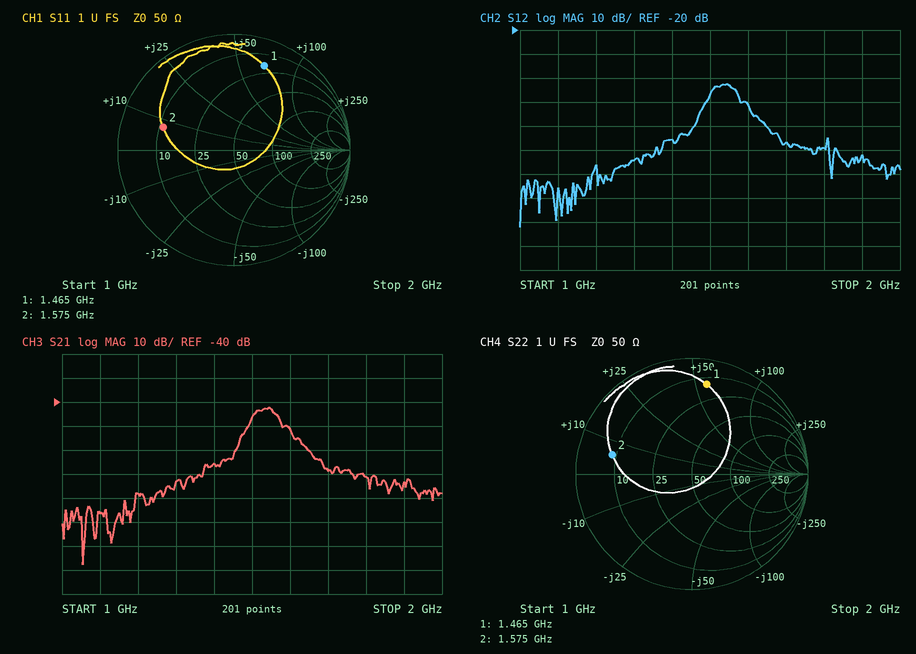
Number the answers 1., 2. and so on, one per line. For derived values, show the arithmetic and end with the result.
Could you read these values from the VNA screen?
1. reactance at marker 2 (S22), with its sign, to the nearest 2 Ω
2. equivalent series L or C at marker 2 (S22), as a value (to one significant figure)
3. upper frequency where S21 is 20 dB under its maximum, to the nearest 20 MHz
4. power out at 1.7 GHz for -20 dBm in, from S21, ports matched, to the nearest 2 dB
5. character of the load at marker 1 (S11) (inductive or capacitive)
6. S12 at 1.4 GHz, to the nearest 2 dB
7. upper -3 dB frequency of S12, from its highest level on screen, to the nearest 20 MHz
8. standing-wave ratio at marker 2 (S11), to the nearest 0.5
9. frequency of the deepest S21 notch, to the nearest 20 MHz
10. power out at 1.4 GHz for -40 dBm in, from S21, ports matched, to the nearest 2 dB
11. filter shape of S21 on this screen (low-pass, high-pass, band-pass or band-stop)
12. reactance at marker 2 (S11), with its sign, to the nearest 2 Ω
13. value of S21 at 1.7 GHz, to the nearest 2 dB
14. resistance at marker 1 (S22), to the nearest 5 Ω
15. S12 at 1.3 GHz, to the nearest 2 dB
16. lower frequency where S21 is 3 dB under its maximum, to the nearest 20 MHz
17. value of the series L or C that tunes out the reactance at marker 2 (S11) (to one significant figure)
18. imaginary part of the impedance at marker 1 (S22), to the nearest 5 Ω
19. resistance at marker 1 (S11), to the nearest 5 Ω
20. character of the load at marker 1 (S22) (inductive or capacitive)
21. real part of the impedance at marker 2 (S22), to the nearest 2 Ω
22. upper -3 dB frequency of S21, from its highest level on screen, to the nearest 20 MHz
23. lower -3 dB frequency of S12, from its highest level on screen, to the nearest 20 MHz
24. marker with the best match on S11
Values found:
1. +6 Ω
2. L = 6 Ω/(2π × 1.575 GHz) ≈ 606 pH, so 600 pH to one significant figure
3. 1.66 GHz
4. -20 dBm + (-68 dB) = -88 dBm
5. inductive
6. -66 dB
7. 1.56 GHz
8. 4.5
9. 1.06 GHz
10. -40 dBm + (-66 dB) = -106 dBm
11. band-pass
12. +8 Ω
13. -68 dB
14. 15 Ω
15. -74 dB
16. 1.50 GHz
17. C = 1/(2π × 1.575 GHz × 8 Ω) ≈ 12.6 pF, so 10 pF to one significant figure
18. +55 Ω
19. 20 Ω
20. inductive
21. 8 Ω
22. 1.56 GHz
23. 1.50 GHz
24. marker 2
